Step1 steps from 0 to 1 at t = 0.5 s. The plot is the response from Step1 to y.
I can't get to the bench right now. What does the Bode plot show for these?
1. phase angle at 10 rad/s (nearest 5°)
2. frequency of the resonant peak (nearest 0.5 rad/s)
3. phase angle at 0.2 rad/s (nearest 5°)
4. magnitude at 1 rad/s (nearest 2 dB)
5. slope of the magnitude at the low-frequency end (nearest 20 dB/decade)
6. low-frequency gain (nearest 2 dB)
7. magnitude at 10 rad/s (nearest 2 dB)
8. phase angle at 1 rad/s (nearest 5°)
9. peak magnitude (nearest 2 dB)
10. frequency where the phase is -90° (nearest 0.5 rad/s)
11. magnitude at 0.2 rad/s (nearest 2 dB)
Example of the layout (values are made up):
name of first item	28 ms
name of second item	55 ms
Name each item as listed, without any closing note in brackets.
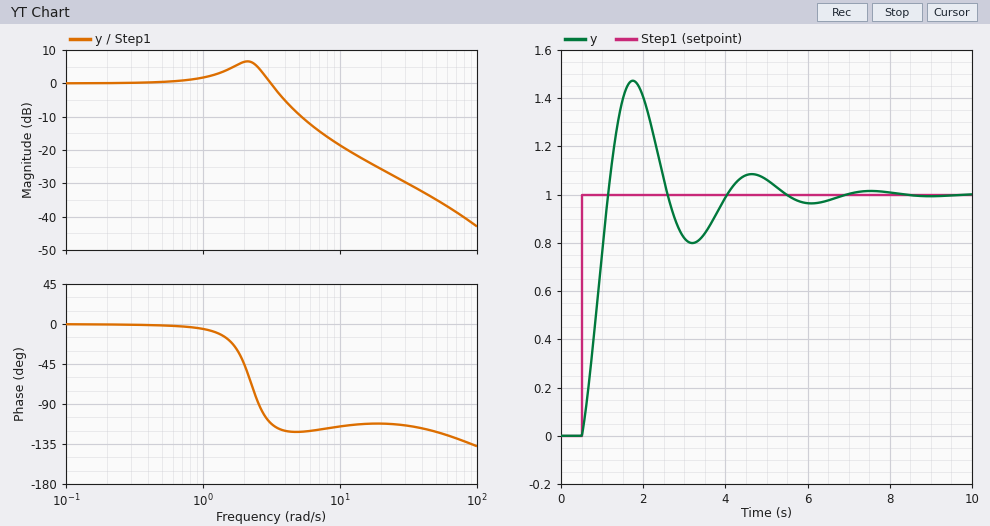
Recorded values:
phase angle at 10 rad/s	-115°
frequency of the resonant peak	2.0 rad/s
phase angle at 0.2 rad/s	0°
magnitude at 1 rad/s	2 dB
slope of the magnitude at the low-frequency end	0 dB/decade
low-frequency gain	0 dB
magnitude at 10 rad/s	-18 dB
phase angle at 1 rad/s	-5°
peak magnitude	6 dB
frequency where the phase is -90°	2.5 rad/s
magnitude at 0.2 rad/s	0 dB
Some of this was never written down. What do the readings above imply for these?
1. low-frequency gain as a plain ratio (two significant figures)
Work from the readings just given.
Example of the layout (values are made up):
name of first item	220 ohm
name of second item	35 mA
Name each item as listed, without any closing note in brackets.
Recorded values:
low-frequency gain as a plain ratio	1.0
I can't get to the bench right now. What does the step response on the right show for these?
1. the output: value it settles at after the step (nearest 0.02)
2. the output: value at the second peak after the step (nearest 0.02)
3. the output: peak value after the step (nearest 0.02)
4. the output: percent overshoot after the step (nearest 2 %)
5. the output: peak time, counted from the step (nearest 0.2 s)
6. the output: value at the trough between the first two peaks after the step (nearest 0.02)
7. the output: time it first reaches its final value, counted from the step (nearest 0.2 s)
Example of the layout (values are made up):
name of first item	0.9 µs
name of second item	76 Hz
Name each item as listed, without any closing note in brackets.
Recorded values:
the output: value it settles at after the step	1.00
the output: value at the second peak after the step	1.08
the output: peak value after the step	1.48
the output: percent overshoot after the step	48 %
the output: peak time, counted from the step	1.2 s
the output: value at the trough between the first two peaks after the step	0.80
the output: time it first reaches its final value, counted from the step	0.6 s
